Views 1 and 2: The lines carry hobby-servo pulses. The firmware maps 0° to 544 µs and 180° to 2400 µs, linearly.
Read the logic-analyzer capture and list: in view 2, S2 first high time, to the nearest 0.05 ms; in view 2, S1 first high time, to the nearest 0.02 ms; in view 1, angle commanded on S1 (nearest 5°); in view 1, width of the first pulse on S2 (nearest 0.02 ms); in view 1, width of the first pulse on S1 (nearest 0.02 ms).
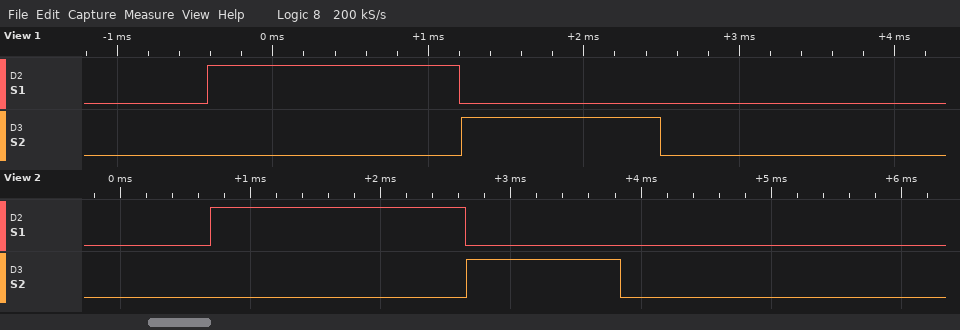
1.20 ms
1.96 ms
105°
1.28 ms
1.62 ms
